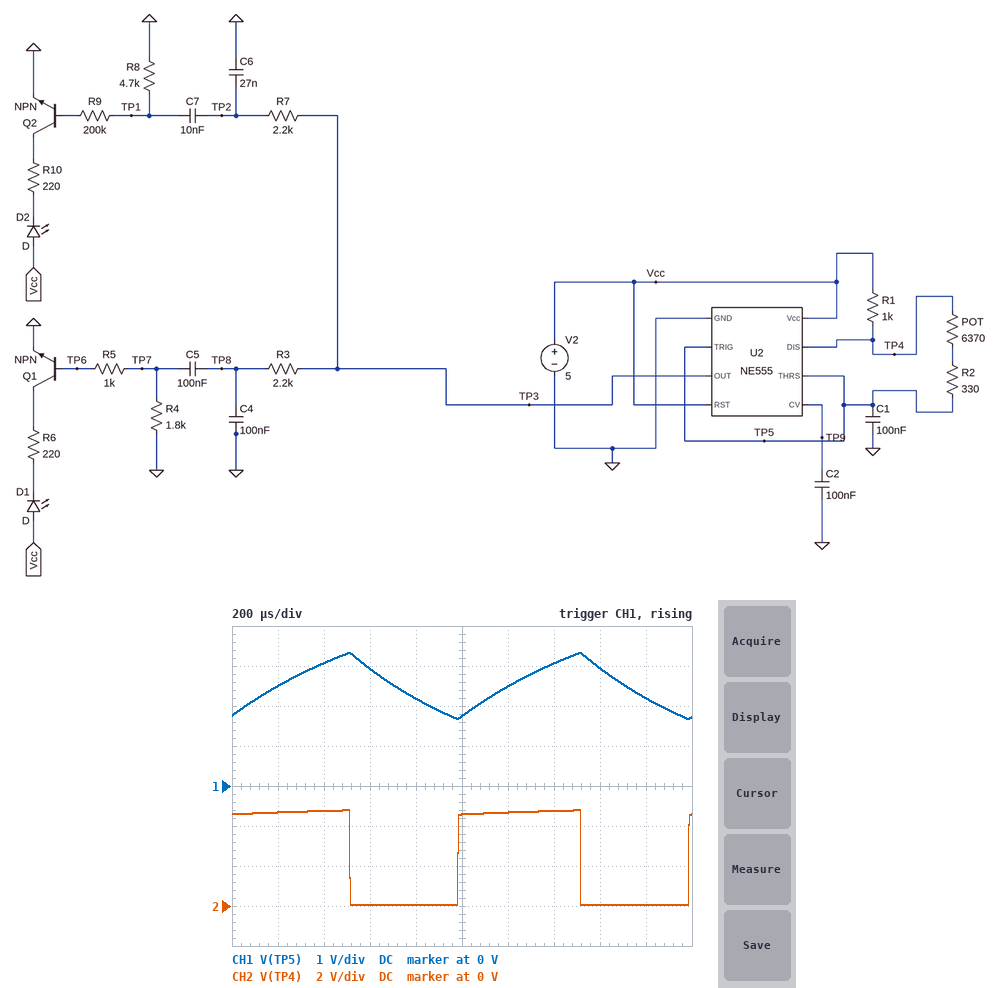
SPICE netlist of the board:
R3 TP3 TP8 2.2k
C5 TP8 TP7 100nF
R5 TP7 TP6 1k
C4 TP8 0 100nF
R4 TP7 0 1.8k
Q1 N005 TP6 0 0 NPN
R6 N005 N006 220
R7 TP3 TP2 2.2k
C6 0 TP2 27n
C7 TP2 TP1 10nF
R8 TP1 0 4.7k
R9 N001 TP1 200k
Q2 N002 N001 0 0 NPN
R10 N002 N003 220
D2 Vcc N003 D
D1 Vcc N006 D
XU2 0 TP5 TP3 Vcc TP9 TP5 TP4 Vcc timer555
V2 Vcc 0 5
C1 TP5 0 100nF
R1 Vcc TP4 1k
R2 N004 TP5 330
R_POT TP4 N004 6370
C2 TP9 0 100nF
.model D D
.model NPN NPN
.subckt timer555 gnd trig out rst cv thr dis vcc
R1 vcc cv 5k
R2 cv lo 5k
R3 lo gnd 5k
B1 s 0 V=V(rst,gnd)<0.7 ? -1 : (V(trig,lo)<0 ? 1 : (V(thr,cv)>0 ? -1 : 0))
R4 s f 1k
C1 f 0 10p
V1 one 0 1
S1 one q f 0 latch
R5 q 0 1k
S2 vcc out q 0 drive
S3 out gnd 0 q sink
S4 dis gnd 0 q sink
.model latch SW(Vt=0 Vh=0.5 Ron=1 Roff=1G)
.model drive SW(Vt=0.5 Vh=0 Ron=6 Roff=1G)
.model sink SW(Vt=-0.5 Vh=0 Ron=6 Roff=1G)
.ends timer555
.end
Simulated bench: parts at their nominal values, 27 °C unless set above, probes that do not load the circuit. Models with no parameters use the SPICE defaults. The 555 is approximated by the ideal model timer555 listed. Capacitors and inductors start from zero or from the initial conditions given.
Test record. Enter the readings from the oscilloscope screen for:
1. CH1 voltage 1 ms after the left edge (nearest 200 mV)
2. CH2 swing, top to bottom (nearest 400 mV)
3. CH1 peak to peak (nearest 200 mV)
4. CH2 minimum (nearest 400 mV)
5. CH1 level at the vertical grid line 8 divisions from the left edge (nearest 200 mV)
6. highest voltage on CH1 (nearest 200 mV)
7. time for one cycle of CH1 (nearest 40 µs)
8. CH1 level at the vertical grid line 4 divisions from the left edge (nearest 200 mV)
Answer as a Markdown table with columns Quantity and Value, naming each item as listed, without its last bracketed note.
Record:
| Quantity | Value |
|---|---|
| CH1 voltage 1 ms after the left edge | 1.8 V |
| CH2 swing, top to bottom | 4.8 V |
| CH1 peak to peak | 1.6 V |
| CH2 minimum | 0 V |
| CH1 level at the vertical grid line 8 divisions from the left edge | 3.0 V |
| highest voltage on CH1 | 3.4 V |
| time for one cycle of CH1 | 1.00 ms |
| CH1 level at the vertical grid line 4 divisions from the left edge | 2.2 V |
